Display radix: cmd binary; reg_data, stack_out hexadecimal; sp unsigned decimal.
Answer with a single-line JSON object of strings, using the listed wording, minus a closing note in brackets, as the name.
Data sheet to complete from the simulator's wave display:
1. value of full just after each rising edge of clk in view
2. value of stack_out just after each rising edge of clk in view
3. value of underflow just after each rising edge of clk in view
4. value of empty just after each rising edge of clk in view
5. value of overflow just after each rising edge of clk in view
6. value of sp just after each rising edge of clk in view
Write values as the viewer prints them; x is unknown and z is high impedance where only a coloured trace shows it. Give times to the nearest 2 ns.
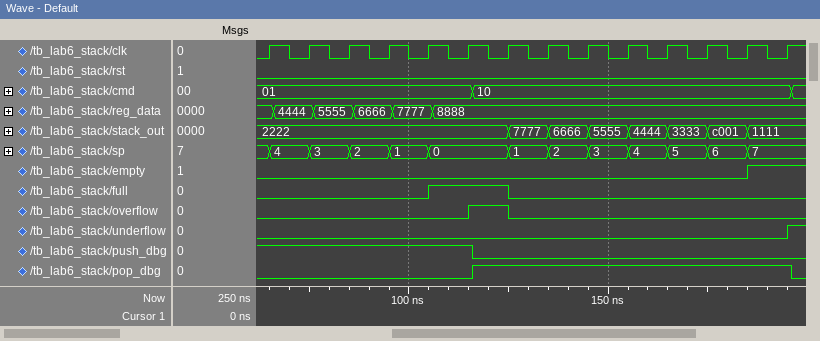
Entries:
{"value of full just after each rising edge of clk in view": "0 0 0 0 1 1 0 0 0 0 0 0 0 0", "value of stack_out just after each rising edge of clk in view": "2222, 2222, 2222, 2222, 2222, 2222, 7777, 6666, 5555, 4444, 3333, c001, 1111, 1111", "value of underflow just after each rising edge of clk in view": "0 0 0 0 0 0 0 0 0 0 0 0 0 1", "value of empty just after each rising edge of clk in view": "0 0 0 0 0 0 0 0 0 0 0 0 1 1", "value of overflow just after each rising edge of clk in view": "0 0 0 0 0 1 0 0 0 0 0 0 0 0", "value of sp just after each rising edge of clk in view": "4, 3, 2, 1, 0, 0, 1, 2, 3, 4, 5, 6, 7, 7"}
